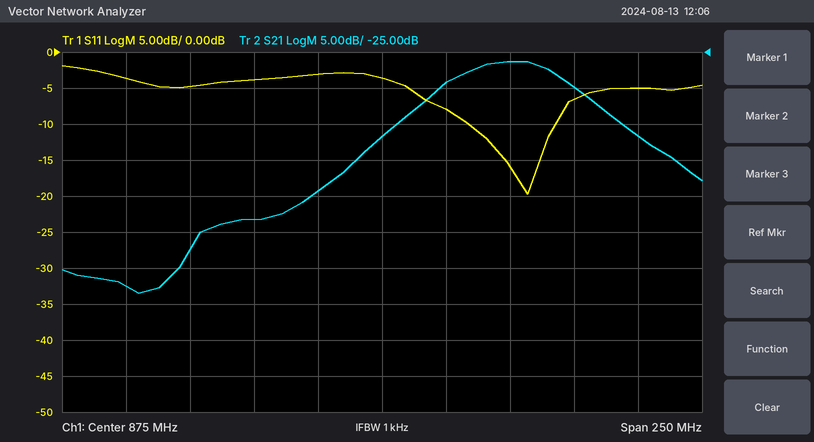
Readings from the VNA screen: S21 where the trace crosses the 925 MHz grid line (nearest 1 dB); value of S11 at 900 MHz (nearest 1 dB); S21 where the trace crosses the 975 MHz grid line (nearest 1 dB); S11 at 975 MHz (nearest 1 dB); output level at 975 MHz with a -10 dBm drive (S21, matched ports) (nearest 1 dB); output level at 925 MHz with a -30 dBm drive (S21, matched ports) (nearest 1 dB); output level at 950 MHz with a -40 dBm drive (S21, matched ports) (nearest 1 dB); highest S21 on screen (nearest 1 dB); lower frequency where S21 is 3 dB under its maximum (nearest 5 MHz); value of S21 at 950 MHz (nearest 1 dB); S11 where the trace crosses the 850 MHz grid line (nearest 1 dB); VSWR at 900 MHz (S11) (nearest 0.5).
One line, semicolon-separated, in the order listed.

-26 dB; -8 dB; -37 dB; -5 dB; -47 dBm; -56 dBm; -70 dBm; -26 dB; 900 MHz; -30 dB; -3 dB; 2.5
